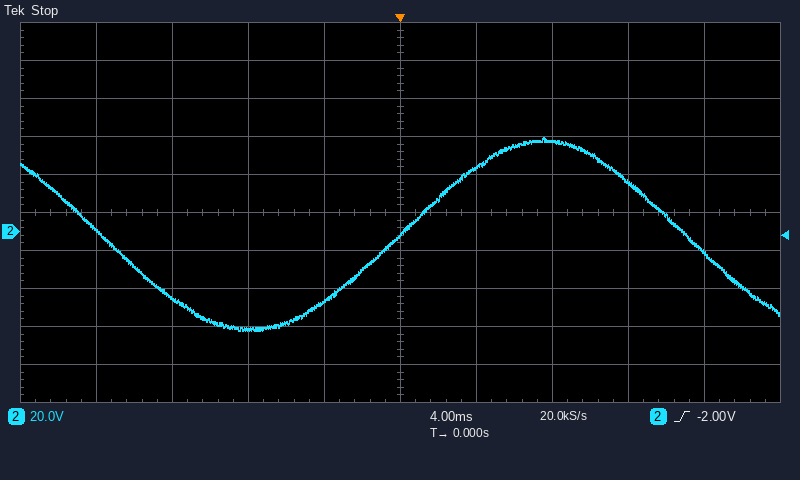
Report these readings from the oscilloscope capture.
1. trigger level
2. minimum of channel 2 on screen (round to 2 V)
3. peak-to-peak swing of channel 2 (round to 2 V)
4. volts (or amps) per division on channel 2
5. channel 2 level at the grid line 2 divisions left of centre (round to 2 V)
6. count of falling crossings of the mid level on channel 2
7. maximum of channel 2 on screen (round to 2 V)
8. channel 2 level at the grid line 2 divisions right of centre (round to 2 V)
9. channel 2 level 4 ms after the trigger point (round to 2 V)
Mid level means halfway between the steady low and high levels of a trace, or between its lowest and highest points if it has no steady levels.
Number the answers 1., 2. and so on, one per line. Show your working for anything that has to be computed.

1. -2.00 V
2. -52 V
3. 50 V − (-52 V) = 102 V
4. 20 V
5. -52 V
6. 2
7. 50 V
8. 48 V
9. 34 V
